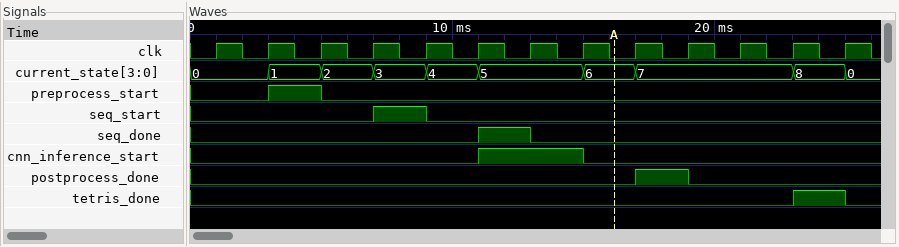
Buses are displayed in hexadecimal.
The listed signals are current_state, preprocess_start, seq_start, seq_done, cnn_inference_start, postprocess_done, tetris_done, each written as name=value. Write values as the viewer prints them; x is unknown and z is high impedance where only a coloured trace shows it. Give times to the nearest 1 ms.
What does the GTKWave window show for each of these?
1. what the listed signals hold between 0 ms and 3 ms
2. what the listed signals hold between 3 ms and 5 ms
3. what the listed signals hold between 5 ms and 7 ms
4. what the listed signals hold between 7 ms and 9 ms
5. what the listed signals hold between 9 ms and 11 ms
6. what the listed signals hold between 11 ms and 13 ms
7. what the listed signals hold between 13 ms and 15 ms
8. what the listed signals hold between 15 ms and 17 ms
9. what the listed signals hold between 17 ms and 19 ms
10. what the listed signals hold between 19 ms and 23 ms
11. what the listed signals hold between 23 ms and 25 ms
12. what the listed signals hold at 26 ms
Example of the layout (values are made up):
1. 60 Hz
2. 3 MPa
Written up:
1. current_state=0, preprocess_start=0, seq_start=0, seq_done=0, cnn_inference_start=0, postprocess_done=0, tetris_done=0
2. current_state=1, preprocess_start=1, seq_start=0, seq_done=0, cnn_inference_start=0, postprocess_done=0, tetris_done=0
3. current_state=2, preprocess_start=0, seq_start=0, seq_done=0, cnn_inference_start=0, postprocess_done=0, tetris_done=0
4. current_state=3, preprocess_start=0, seq_start=1, seq_done=0, cnn_inference_start=0, postprocess_done=0, tetris_done=0
5. current_state=4, preprocess_start=0, seq_start=0, seq_done=0, cnn_inference_start=0, postprocess_done=0, tetris_done=0
6. current_state=5, preprocess_start=0, seq_start=0, seq_done=1, cnn_inference_start=1, postprocess_done=0, tetris_done=0
7. current_state=5, preprocess_start=0, seq_start=0, seq_done=0, cnn_inference_start=1, postprocess_done=0, tetris_done=0
8. current_state=6, preprocess_start=0, seq_start=0, seq_done=0, cnn_inference_start=0, postprocess_done=0, tetris_done=0
9. current_state=7, preprocess_start=0, seq_start=0, seq_done=0, cnn_inference_start=0, postprocess_done=1, tetris_done=0
10. current_state=7, preprocess_start=0, seq_start=0, seq_done=0, cnn_inference_start=0, postprocess_done=0, tetris_done=0
11. current_state=8, preprocess_start=0, seq_start=0, seq_done=0, cnn_inference_start=0, postprocess_done=0, tetris_done=1
12. current_state=0, preprocess_start=0, seq_start=0, seq_done=0, cnn_inference_start=0, postprocess_done=0, tetris_done=0
